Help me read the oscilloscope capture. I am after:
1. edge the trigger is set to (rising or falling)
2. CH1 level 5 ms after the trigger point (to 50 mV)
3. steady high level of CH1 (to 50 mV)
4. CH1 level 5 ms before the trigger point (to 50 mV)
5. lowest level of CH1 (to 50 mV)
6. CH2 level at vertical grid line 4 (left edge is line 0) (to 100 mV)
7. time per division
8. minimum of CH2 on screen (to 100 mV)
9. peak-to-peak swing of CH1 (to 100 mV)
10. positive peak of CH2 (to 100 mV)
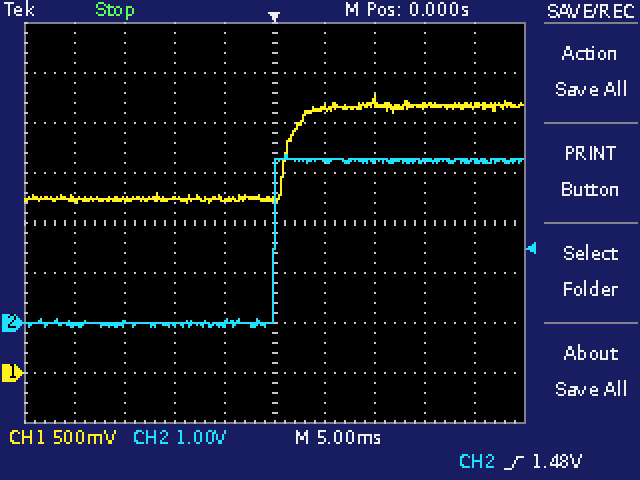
rising
2.65 V
2.65 V
1.75 V
1.70 V
0.0 V
5 ms
-100 mV
1.10 V
3.4 V
